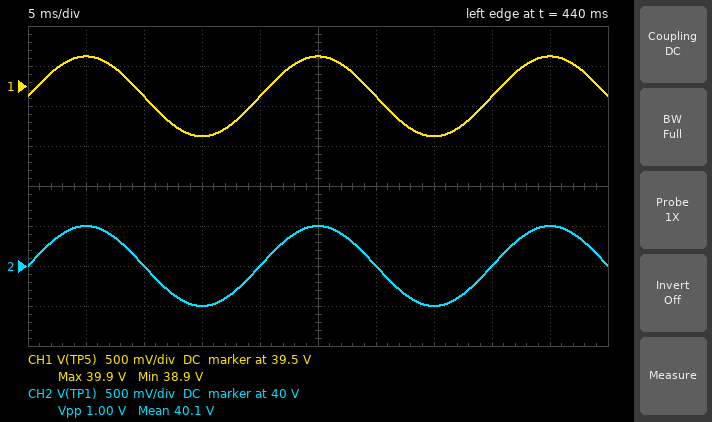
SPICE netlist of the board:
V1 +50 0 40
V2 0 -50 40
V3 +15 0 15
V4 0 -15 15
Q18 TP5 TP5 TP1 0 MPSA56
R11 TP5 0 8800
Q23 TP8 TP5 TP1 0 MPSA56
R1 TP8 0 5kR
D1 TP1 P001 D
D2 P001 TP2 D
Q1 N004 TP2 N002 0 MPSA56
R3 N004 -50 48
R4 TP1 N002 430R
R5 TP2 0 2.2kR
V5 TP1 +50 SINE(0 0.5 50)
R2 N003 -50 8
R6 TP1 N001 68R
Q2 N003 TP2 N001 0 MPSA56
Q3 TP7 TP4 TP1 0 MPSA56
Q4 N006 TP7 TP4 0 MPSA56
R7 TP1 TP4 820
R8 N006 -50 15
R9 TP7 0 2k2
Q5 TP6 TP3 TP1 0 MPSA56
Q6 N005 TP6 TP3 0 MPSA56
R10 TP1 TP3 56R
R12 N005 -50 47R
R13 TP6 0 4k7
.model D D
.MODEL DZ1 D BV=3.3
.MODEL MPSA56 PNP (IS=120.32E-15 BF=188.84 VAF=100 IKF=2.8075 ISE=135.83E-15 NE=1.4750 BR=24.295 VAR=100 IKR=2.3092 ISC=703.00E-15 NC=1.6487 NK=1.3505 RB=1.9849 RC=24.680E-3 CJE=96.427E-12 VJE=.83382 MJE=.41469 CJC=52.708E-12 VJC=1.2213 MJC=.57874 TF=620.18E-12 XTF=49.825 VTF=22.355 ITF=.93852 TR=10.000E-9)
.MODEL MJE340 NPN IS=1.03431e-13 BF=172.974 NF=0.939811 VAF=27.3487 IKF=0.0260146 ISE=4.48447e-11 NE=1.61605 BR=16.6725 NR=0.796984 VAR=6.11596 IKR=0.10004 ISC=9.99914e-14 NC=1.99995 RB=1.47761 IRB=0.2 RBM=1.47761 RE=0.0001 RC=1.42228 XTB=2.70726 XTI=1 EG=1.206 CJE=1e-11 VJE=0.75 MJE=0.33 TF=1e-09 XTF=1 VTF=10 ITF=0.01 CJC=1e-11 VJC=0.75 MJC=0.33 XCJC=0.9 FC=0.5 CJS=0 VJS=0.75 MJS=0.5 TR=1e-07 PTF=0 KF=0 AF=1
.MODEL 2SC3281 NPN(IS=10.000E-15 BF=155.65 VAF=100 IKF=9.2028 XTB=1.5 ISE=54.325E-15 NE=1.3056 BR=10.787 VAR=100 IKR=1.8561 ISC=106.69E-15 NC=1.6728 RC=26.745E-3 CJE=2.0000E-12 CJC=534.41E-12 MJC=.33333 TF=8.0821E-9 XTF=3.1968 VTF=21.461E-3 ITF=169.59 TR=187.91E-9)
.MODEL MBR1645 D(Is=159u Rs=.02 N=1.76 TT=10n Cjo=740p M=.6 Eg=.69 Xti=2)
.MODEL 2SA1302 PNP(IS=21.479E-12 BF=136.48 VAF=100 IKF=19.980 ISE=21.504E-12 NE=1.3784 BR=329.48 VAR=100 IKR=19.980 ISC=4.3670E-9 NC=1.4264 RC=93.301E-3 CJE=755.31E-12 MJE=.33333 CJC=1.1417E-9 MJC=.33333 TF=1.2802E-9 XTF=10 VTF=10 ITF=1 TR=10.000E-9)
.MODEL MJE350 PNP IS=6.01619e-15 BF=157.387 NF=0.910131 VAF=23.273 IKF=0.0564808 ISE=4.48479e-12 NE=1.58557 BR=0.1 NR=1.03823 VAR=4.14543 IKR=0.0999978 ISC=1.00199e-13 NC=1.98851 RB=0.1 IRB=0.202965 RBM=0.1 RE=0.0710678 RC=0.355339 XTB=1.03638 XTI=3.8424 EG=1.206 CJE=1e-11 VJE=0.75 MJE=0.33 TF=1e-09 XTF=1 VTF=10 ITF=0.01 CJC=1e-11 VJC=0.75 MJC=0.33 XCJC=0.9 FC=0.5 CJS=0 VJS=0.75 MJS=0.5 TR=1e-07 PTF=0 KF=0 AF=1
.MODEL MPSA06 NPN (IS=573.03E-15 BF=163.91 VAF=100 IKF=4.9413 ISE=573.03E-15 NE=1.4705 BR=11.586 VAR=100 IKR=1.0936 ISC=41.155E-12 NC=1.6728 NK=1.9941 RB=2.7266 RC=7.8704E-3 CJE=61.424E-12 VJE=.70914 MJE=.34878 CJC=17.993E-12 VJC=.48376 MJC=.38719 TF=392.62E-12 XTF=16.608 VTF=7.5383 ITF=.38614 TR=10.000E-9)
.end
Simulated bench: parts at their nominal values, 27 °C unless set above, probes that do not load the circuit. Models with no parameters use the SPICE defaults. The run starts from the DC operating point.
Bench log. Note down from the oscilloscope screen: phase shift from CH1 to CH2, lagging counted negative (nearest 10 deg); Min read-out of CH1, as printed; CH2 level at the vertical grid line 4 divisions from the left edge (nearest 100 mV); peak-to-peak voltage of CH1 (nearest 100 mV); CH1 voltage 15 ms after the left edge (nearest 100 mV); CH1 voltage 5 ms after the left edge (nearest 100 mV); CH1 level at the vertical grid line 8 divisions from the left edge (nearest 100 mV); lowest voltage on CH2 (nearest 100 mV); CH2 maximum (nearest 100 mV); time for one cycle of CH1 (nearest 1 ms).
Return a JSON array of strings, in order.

["0 deg", "38.9 V", "40.0 V", "1.0 V", "38.9 V", "39.9 V", "39.4 V", "39.5 V", "40.5 V", "20 ms"]
